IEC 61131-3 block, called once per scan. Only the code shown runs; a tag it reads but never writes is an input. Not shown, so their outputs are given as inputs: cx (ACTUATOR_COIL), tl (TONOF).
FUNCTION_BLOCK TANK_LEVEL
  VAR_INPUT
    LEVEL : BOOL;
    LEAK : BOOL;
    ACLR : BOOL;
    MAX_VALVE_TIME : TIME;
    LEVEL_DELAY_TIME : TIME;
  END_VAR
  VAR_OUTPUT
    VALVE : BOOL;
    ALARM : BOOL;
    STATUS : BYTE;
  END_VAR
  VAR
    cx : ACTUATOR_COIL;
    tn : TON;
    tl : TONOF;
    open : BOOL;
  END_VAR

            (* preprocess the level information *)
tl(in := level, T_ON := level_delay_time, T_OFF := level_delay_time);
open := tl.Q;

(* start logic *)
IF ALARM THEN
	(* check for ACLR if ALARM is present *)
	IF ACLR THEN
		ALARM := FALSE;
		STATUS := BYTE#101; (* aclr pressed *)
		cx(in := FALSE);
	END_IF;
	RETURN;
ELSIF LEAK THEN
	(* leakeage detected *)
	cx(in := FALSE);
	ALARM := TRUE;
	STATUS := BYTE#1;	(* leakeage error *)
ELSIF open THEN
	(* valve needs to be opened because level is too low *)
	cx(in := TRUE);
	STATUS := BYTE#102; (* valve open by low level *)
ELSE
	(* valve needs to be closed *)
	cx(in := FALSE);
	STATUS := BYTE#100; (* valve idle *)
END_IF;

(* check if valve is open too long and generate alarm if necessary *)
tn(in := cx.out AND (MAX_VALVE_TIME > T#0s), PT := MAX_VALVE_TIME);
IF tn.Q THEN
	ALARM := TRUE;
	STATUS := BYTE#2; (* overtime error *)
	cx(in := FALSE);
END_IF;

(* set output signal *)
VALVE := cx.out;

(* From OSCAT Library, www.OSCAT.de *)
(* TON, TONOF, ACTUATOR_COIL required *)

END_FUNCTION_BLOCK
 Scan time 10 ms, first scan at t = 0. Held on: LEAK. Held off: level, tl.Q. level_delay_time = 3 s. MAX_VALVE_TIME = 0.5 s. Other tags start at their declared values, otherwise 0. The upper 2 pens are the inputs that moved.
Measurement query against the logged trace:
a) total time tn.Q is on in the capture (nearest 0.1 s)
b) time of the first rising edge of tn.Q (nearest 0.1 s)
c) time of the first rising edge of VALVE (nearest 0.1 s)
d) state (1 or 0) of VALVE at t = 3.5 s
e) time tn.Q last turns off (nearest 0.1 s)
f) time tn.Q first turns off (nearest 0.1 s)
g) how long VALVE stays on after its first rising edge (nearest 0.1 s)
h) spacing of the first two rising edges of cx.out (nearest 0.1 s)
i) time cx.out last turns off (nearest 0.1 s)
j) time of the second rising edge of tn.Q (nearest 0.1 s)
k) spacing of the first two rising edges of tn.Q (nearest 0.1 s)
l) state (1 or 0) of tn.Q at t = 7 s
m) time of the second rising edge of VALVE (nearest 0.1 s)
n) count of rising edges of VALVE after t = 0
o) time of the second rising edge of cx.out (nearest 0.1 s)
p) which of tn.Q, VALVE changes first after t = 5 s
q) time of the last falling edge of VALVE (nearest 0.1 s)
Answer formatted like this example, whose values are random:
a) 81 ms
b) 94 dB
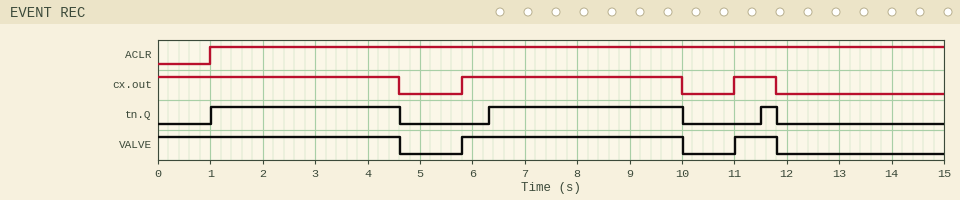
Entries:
a) 7.6 s
b) 1.0 s
c) 5.8 s
d) 1
e) 11.8 s
f) 4.6 s
g) 4.2 s
h) 5.2 s
i) 11.8 s
j) 6.3 s
k) 5.3 s
l) 1
m) 11.0 s
n) 2
o) 11.0 s
p) VALVE
q) 11.8 s
